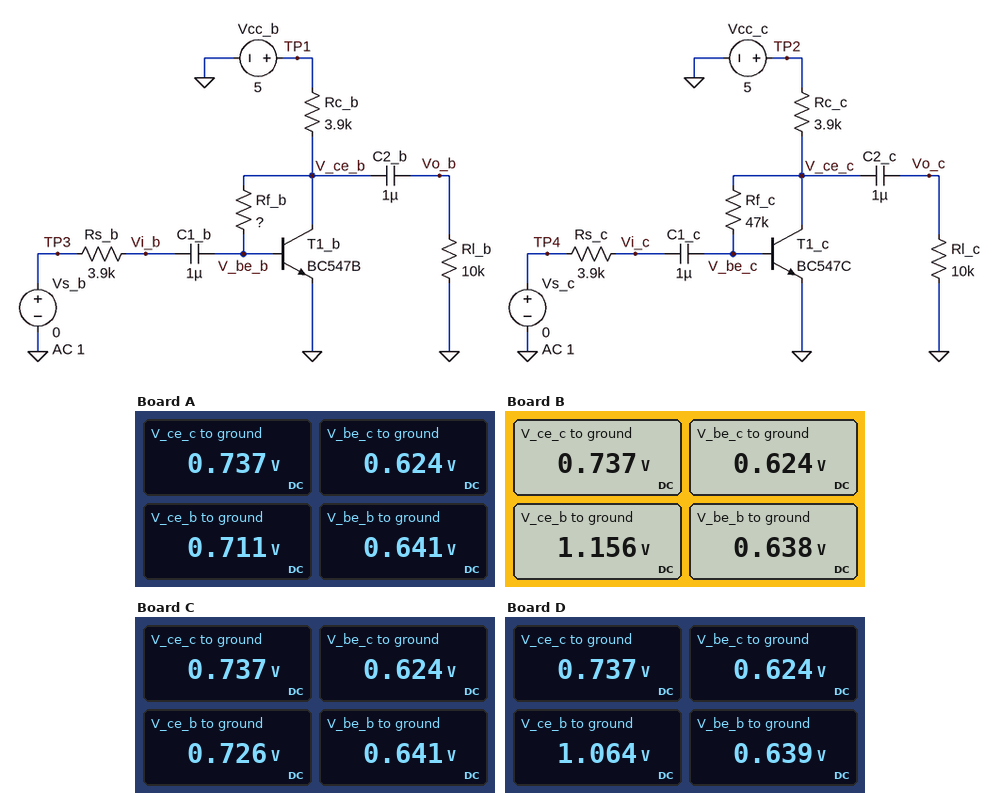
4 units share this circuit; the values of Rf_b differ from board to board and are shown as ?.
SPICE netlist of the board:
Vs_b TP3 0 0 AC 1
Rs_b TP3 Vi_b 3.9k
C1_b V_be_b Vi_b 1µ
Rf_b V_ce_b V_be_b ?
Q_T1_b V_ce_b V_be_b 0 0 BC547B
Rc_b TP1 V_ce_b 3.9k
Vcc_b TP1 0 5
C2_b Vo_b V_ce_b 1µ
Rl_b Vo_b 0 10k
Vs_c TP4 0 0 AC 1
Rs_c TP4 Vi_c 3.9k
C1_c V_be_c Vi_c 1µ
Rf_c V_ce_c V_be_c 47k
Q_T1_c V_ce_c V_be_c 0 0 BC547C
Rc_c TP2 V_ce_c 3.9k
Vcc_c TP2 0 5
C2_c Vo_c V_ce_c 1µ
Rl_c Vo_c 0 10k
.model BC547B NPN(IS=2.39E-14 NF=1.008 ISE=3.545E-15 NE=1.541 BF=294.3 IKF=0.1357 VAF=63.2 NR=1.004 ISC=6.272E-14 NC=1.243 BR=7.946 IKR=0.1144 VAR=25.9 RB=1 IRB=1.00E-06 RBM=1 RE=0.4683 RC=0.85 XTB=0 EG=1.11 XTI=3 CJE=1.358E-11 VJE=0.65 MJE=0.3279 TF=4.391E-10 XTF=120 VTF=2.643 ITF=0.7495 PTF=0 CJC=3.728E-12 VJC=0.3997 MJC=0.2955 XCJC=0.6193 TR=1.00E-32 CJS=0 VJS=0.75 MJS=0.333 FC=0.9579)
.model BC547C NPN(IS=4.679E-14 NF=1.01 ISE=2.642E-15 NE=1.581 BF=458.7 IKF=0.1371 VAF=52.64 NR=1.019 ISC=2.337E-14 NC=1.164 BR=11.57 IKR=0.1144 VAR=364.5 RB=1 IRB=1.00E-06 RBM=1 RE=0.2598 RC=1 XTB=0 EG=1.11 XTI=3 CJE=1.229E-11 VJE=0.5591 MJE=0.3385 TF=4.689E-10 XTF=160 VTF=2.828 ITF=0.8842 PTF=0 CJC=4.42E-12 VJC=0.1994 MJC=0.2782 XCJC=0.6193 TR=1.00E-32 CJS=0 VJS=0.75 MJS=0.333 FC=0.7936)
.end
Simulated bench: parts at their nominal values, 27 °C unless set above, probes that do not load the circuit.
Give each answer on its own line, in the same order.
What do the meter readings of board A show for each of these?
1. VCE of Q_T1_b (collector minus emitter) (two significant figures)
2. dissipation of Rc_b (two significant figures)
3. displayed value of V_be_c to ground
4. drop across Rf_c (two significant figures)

710 mV
4.7 mW
0.624 V
110 mV
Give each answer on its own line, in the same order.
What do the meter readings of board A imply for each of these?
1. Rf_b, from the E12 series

18 kΩ
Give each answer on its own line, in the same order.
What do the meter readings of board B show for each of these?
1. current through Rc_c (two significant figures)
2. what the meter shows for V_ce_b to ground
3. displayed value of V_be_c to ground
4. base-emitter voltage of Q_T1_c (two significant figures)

1.1 mA
1.156 V
0.624 V
620 mV
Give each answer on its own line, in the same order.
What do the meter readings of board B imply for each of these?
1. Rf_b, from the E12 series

150 kΩ
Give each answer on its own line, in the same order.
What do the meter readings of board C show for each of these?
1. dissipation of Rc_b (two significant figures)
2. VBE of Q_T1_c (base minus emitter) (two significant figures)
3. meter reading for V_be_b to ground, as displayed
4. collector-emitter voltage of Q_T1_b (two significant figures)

4.7 mW
620 mV
0.641 V
730 mV
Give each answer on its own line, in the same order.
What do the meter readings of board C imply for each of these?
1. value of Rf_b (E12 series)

22 kΩ
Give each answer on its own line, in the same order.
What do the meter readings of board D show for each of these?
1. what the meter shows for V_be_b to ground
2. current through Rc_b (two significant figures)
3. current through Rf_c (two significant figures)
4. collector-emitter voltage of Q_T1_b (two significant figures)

0.639 V
1.0 mA
2.4 µA
1.1 V
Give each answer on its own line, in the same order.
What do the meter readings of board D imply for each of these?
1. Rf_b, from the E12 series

120 kΩ
